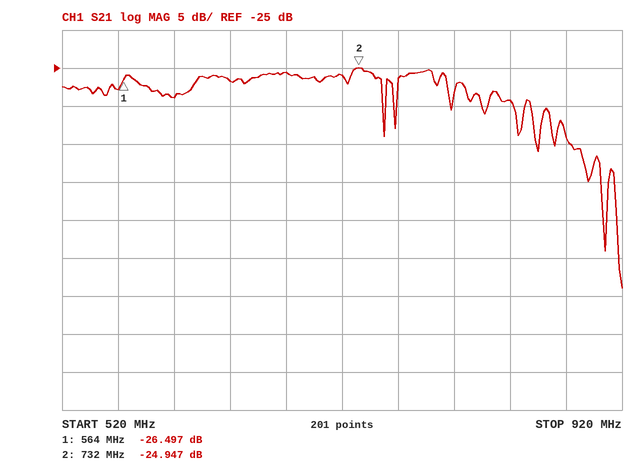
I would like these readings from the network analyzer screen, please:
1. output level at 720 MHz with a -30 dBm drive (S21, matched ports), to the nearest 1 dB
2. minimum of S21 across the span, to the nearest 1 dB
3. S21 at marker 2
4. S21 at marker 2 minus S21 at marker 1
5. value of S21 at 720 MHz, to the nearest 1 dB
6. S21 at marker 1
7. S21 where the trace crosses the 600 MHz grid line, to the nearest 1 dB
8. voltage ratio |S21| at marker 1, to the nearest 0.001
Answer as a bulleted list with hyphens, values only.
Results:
- -56 dBm
- -54 dB
- -24.947 dB
- 1.550 dB
- -26 dB
- -26.497 dB
- -29 dB
- 0.047
